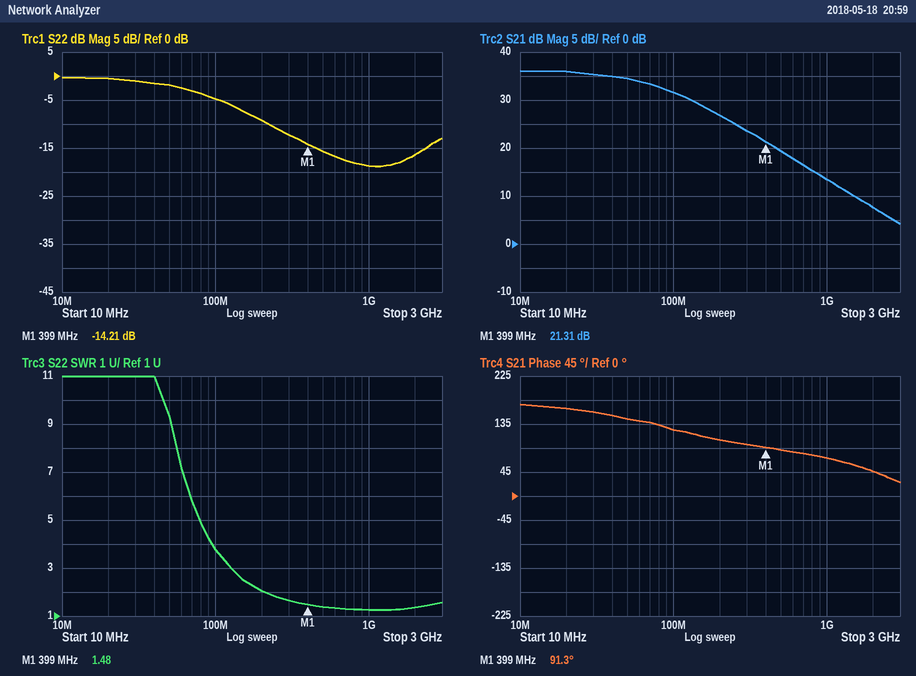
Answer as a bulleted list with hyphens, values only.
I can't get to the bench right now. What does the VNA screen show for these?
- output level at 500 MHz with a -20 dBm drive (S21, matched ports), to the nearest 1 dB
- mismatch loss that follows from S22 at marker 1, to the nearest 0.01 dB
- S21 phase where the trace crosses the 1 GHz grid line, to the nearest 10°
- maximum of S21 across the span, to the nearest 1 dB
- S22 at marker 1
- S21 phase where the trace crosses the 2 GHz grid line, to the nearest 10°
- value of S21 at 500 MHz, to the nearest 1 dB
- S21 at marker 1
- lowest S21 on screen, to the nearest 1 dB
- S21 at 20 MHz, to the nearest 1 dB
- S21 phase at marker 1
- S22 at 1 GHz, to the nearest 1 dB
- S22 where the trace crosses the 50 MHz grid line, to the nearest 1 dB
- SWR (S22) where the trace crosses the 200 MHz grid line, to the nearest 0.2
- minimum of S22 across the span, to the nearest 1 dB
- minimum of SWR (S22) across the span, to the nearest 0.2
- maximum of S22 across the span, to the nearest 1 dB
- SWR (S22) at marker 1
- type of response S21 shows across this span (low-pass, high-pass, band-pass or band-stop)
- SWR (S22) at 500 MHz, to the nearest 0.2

- -1 dBm
- 0.17 dB
- 70°
- 36 dB
- -14.21 dB
- 50°
- 19 dB
- 21.31 dB
- 4 dB
- 36 dB
- 91.3°
- -19 dB
- -2 dB
- 2.0
- -19 dB
- 1.2
- 0 dB
- 1.48
- low-pass
- 1.4
